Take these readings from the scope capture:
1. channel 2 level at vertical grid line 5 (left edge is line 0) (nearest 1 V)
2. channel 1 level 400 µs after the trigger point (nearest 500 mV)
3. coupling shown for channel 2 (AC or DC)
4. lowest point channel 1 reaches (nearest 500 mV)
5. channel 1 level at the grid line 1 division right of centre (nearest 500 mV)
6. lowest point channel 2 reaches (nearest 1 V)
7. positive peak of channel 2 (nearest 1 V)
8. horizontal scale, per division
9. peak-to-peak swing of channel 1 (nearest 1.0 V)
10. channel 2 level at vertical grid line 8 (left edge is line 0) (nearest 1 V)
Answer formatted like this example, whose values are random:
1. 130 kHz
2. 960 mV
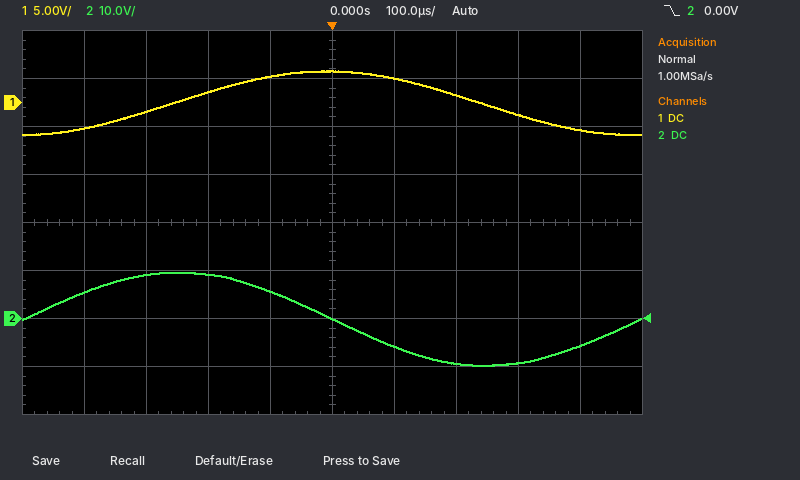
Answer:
1. 0 V
2. -3.0 V
3. DC
4. -3.5 V
5. 2.5 V
6. -10 V
7. 10 V
8. 100 µs
9. 7.0 V
10. -9 V
